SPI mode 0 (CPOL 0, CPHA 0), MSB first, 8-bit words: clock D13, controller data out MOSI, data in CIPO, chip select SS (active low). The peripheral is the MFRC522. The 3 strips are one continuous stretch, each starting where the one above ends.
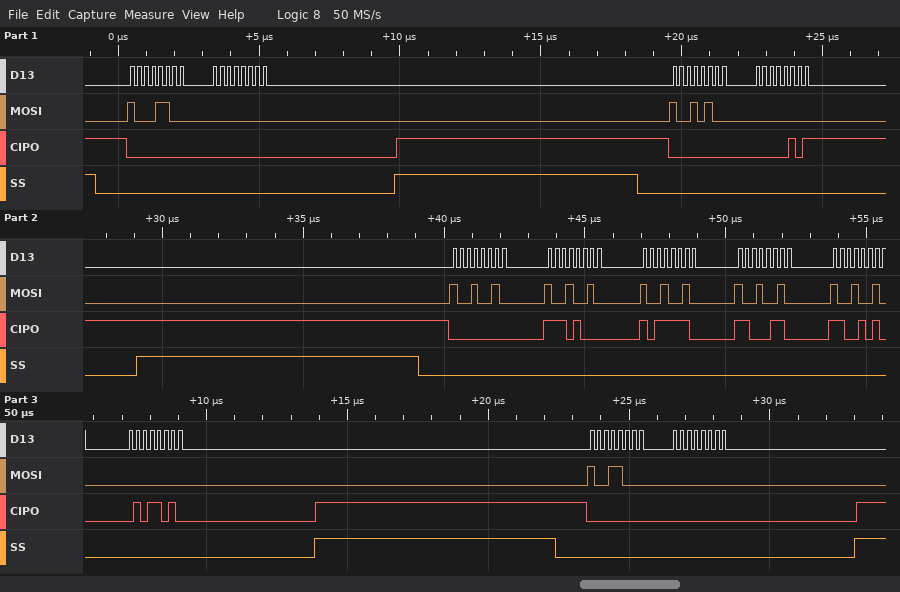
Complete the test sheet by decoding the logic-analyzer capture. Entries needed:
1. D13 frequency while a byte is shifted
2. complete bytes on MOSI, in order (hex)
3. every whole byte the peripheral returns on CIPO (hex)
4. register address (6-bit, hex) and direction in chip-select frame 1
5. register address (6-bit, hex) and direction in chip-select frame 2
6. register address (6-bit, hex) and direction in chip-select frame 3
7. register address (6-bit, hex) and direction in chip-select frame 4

4 MHz
0x8C 0x00 0x94 0x00 0x92 0x92 0x92 0x92 0x92 0x00 0x98 0x00
0x00 0x00 0x00 0x05 0x00 0xE8 0xBE 0xC6 0xCA 0x5A 0x00 0x00
0x06 read
0x0A read
0x09 read
0x0C read
